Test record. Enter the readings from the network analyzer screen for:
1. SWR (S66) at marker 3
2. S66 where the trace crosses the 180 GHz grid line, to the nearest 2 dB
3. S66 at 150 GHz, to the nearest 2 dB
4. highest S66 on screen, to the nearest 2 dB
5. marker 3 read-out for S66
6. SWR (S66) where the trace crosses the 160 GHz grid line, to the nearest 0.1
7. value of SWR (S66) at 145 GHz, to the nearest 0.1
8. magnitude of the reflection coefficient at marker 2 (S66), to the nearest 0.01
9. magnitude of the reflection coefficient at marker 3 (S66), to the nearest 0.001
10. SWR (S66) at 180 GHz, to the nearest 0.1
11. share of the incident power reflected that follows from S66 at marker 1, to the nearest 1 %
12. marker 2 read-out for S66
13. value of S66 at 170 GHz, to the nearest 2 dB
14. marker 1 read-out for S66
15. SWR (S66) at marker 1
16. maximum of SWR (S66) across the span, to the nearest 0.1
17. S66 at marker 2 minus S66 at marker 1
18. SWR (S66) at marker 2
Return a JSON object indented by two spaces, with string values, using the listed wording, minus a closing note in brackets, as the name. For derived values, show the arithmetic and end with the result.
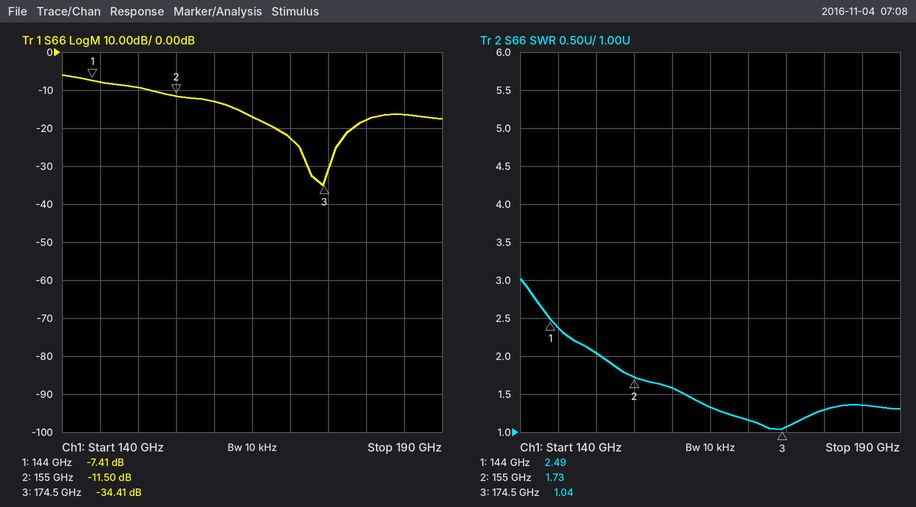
{
  "SWR (S66) at marker 3": "1.04",
  "S66 where the trace crosses the 180 GHz grid line, to the nearest 2 dB": "-18 dB",
  "S66 at 150 GHz, to the nearest 2 dB": "-10 dB",
  "highest S66 on screen, to the nearest 2 dB": "-6 dB",
  "marker 3 read-out for S66": "-34.41 dB",
  "SWR (S66) where the trace crosses the 160 GHz grid line, to the nearest 0.1": "1.6",
  "value of SWR (S66) at 145 GHz, to the nearest 0.1": "2.4",
  "magnitude of the reflection coefficient at marker 2 (S66), to the nearest 0.01": "10^(-11.5/20) ≈ 0.27",
  "magnitude of the reflection coefficient at marker 3 (S66), to the nearest 0.001": "10^(-34.41/20) ≈ 0.019",
  "SWR (S66) at 180 GHz, to the nearest 0.1": "1.3",
  "share of the incident power reflected that follows from S66 at marker 1, to the nearest 1 %": "10^(-7.41/10) ≈ 18 %",
  "marker 2 read-out for S66": "-11.50 dB",
  "value of S66 at 170 GHz, to the nearest 2 dB": "-22 dB",
  "marker 1 read-out for S66": "-7.41 dB",
  "SWR (S66) at marker 1": "2.49",
  "maximum of SWR (S66) across the span, to the nearest 0.1": "3.0",
  "S66 at marker 2 minus S66 at marker 1": "-11.5 − (-7.41) = -4.09 dB",
  "SWR (S66) at marker 2": "1.73"
}
